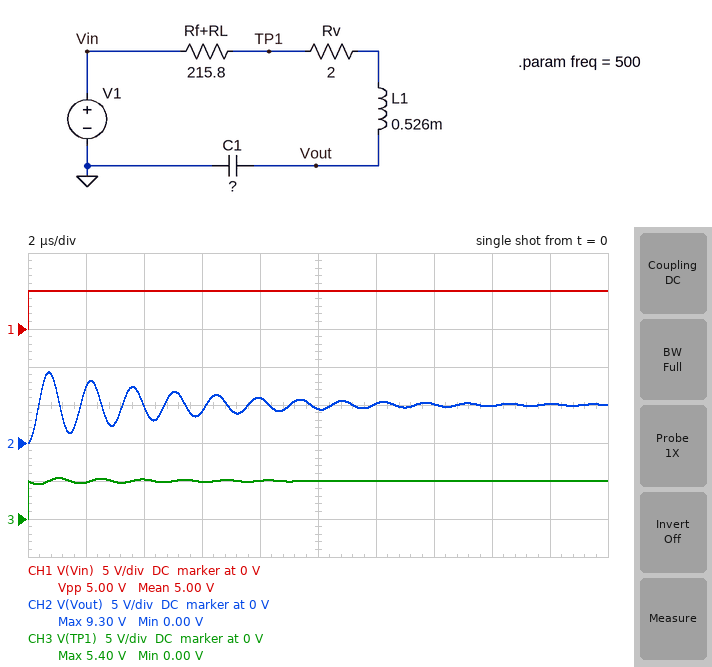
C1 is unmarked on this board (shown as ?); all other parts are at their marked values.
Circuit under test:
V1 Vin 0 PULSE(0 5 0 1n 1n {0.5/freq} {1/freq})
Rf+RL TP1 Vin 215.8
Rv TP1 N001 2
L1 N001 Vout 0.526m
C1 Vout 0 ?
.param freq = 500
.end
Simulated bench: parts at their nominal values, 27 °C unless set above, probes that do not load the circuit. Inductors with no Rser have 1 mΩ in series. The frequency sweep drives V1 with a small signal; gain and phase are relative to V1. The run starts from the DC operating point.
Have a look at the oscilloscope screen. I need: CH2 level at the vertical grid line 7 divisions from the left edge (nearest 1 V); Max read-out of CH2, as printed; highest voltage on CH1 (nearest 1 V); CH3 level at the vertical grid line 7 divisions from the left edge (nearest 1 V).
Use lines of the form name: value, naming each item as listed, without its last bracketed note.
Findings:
CH2 level at the vertical grid line 7 divisions from the left edge: 5 V
Max read-out of CH2, as printed: 9.30 V
highest voltage on CH1: 5 V
CH3 level at the vertical grid line 7 divisions from the left edge: 5 V
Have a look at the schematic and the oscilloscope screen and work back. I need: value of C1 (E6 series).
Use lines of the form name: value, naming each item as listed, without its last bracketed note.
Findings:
value of C1: 100 pF
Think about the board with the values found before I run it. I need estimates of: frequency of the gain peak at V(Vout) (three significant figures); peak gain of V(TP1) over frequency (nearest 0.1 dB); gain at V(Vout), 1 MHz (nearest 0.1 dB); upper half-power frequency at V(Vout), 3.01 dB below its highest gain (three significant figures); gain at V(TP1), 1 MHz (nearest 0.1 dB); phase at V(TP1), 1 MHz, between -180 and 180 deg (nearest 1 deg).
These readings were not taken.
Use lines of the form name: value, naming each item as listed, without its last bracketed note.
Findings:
frequency of the gain peak at V(Vout): 692 kHz
peak gain of V(TP1) over frequency: 0 dB
gain at V(Vout), 1 MHz: -0.7 dB
upper half-power frequency at V(Vout), 3.01 dB below its highest gain: 725 kHz
gain at V(TP1), 1 MHz: -0.1 dB
phase at V(TP1), 1 MHz, between -180 and 180 deg: 7 deg
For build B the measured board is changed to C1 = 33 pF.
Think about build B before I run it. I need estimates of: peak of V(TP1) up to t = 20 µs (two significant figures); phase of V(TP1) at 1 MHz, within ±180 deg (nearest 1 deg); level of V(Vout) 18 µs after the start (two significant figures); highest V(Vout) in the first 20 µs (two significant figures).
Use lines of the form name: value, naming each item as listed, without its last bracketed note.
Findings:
peak of V(TP1) up to t = 20 µs: 5.2 V
phase of V(TP1) at 1 MHz, within ±180 deg: -8 deg
level of V(Vout) 18 µs after the start: 5.0 V
highest V(Vout) in the first 20 µs: 9.6 V
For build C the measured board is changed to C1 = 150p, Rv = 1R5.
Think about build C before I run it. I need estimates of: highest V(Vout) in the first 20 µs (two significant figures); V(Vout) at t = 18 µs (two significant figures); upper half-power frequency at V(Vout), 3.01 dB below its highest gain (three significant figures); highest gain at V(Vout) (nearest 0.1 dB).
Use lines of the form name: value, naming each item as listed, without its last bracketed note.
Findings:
highest V(Vout) in the first 20 µs: 9.2 V
V(Vout) at t = 18 µs: 4.9 V
upper half-power frequency at V(Vout), 3.01 dB below its highest gain: 597 kHz
highest gain at V(Vout): 18.7 dB
